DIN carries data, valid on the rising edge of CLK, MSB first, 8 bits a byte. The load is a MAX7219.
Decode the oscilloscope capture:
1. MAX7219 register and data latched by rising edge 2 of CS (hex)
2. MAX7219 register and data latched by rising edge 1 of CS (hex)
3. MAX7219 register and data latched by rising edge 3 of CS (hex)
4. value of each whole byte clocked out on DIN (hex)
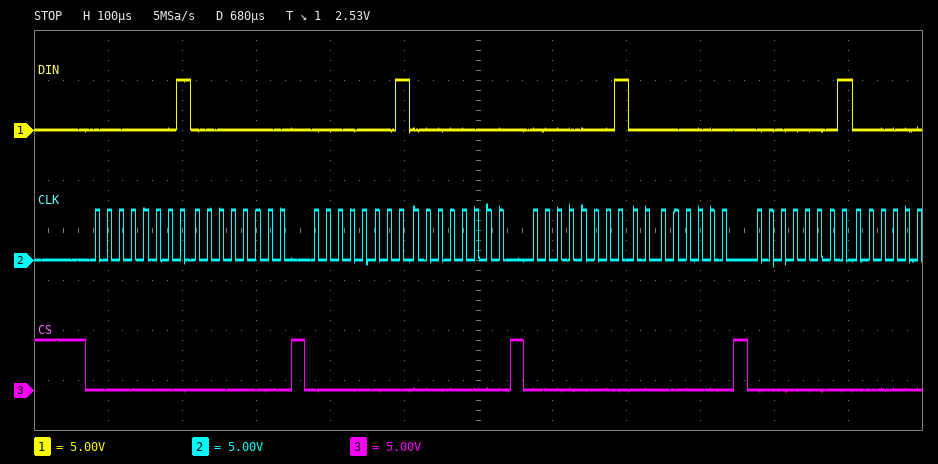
register 0x1, data 0x00
register 0x1, data 0x00
register 0x1, data 0x00
01 00 01 00 01 00 01
